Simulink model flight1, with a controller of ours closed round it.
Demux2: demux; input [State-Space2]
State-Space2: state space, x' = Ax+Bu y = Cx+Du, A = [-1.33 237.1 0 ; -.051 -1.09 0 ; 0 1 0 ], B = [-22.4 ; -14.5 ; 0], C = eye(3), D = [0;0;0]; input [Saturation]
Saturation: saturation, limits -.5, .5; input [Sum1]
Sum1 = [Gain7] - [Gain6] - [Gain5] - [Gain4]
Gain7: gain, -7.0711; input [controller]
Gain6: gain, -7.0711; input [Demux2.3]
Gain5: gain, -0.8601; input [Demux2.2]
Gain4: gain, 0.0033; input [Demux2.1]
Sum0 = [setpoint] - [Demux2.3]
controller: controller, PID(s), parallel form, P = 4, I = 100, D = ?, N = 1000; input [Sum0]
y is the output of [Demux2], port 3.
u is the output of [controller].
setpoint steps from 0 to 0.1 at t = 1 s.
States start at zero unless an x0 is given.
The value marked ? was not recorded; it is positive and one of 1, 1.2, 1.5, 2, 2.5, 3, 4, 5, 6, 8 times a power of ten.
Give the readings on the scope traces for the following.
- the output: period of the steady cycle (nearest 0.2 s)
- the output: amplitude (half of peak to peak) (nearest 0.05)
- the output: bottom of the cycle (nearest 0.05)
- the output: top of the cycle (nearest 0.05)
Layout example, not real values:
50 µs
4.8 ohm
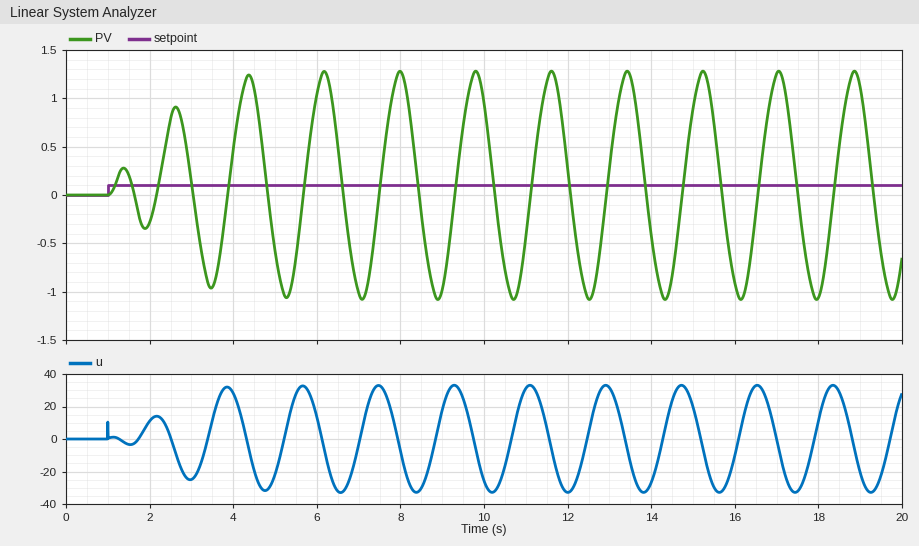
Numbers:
1.8 s
1.20
-1.10
1.30
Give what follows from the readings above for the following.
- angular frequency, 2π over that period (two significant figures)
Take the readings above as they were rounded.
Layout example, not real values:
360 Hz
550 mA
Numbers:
3.5 rad/s
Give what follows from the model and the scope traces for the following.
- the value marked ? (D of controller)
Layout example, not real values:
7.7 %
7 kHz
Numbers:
0.1
